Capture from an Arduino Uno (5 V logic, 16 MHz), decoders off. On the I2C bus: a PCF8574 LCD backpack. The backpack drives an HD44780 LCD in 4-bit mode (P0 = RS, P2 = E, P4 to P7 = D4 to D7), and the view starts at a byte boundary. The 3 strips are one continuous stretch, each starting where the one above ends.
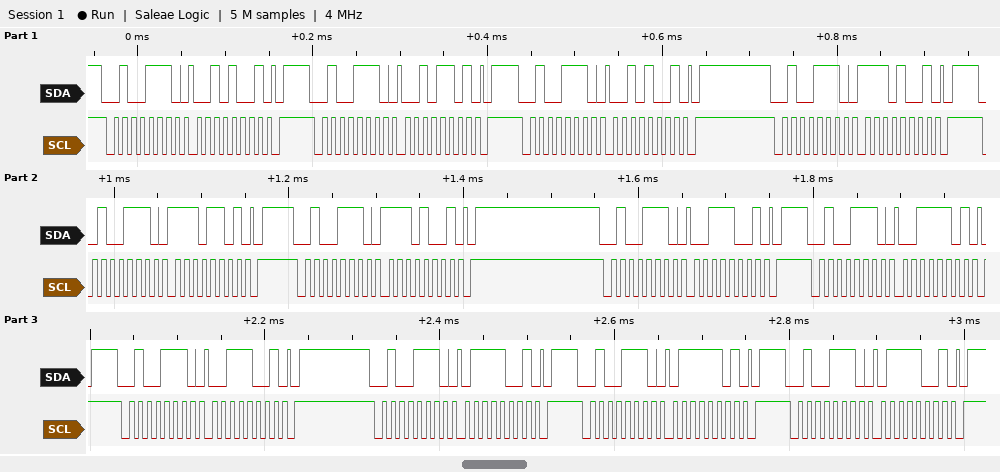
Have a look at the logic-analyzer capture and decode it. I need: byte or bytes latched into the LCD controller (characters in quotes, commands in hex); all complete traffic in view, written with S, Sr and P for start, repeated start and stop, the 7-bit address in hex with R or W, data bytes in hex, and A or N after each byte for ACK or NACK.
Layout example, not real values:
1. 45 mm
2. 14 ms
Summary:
1. '.' '7'
2. S 27W A 29 A P S 27W A 2D A P S 27W A 29 A P S 27W A E9 A P S 27W A ED A P S 27W A E9 A P S 27W A 39 A P S 27W A 3D A P S 27W A 39 A P S 27W A 79 A P S 27W A 7D A P S 27W A 79 A P
